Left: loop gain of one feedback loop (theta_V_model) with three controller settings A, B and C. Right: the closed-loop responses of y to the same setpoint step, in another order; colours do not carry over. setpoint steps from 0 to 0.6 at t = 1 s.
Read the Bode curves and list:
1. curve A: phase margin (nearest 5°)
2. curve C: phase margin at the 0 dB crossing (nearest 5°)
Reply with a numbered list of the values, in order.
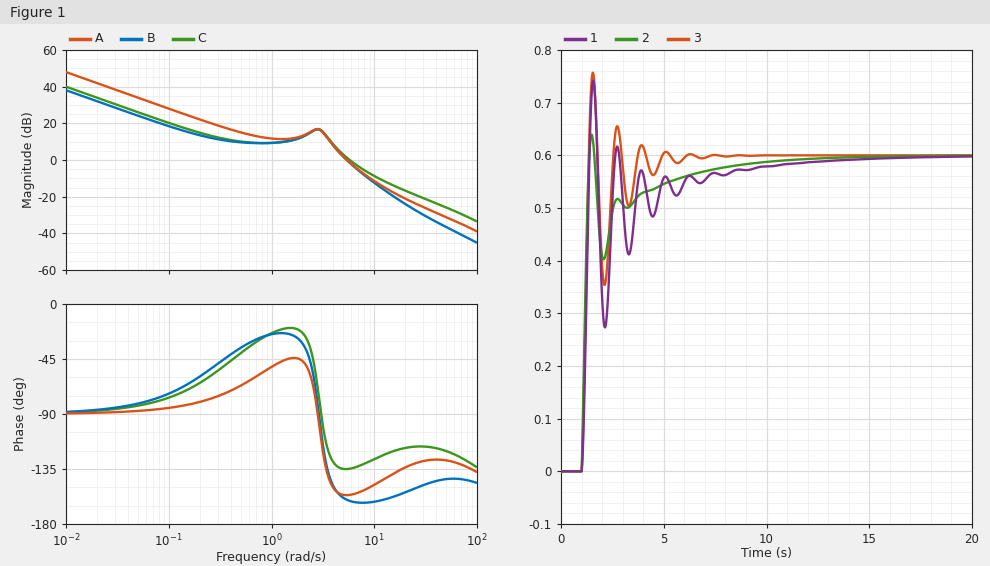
1. 25°
2. 45°
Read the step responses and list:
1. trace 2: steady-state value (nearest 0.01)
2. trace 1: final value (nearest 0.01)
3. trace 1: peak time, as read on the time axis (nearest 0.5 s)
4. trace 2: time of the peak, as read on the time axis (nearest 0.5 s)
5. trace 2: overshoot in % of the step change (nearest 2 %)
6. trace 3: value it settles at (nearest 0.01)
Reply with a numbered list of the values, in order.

1. 0.60
2. 0.60
3. 1.5 s
4. 1.5 s
5. 6 %
6. 0.60
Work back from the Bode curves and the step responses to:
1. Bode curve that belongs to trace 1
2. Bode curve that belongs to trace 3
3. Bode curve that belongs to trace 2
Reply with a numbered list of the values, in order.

1. B
2. A
3. C
